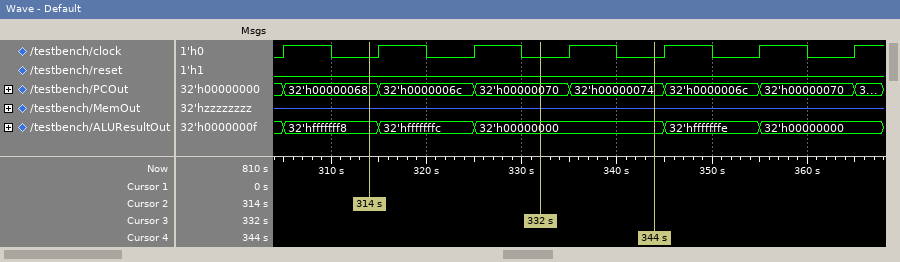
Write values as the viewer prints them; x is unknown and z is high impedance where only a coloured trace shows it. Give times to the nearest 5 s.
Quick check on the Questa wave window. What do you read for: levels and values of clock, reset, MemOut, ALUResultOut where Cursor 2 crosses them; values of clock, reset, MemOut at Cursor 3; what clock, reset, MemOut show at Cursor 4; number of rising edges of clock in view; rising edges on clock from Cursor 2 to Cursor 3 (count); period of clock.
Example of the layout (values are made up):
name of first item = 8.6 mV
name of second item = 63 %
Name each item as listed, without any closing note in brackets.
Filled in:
levels and values of clock, reset, MemOut, ALUResultOut where Cursor 2 crosses them = clock=0, reset=0, MemOut=z, ALUResultOut=32'hfffffff8
values of clock, reset, MemOut at Cursor 3 = clock=0, reset=0, MemOut=z
what clock, reset, MemOut show at Cursor 4 = clock=0, reset=0, MemOut=z
number of rising edges of clock in view = 7
rising edges on clock from Cursor 2 to Cursor 3 = 2
period of clock = 10 s
